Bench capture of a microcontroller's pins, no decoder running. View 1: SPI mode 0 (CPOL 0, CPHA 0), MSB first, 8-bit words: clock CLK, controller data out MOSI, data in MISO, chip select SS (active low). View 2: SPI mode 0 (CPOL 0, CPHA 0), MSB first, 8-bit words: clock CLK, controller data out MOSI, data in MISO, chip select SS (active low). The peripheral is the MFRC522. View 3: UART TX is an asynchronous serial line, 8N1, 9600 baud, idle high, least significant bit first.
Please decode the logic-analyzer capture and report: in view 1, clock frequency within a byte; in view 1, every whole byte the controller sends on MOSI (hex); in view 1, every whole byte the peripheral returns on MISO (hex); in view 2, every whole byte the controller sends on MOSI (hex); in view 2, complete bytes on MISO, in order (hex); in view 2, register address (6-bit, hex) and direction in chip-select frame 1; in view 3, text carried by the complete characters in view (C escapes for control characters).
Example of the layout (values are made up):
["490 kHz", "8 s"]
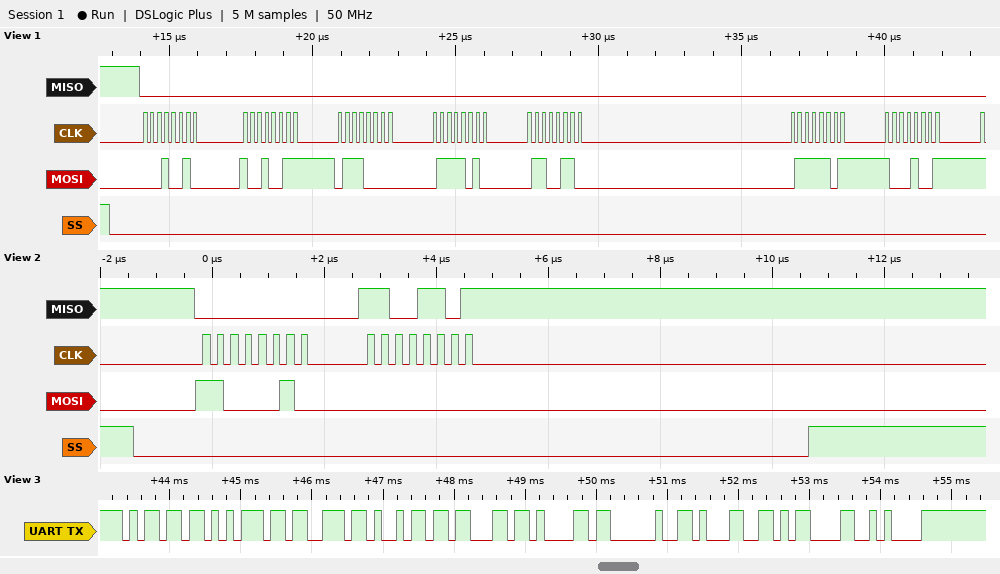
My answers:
["4 MHz", "0x12 0x93 0x70 0x7A 0x66 0x7D 0x89", "0x00 0x00 0x00 0x00 0x00 0x00 0x00", "0xC2 0x00", "0x00 0xCD", "0x21 read", "\"musica 1\\r\\n\""]
